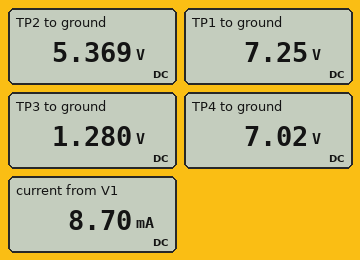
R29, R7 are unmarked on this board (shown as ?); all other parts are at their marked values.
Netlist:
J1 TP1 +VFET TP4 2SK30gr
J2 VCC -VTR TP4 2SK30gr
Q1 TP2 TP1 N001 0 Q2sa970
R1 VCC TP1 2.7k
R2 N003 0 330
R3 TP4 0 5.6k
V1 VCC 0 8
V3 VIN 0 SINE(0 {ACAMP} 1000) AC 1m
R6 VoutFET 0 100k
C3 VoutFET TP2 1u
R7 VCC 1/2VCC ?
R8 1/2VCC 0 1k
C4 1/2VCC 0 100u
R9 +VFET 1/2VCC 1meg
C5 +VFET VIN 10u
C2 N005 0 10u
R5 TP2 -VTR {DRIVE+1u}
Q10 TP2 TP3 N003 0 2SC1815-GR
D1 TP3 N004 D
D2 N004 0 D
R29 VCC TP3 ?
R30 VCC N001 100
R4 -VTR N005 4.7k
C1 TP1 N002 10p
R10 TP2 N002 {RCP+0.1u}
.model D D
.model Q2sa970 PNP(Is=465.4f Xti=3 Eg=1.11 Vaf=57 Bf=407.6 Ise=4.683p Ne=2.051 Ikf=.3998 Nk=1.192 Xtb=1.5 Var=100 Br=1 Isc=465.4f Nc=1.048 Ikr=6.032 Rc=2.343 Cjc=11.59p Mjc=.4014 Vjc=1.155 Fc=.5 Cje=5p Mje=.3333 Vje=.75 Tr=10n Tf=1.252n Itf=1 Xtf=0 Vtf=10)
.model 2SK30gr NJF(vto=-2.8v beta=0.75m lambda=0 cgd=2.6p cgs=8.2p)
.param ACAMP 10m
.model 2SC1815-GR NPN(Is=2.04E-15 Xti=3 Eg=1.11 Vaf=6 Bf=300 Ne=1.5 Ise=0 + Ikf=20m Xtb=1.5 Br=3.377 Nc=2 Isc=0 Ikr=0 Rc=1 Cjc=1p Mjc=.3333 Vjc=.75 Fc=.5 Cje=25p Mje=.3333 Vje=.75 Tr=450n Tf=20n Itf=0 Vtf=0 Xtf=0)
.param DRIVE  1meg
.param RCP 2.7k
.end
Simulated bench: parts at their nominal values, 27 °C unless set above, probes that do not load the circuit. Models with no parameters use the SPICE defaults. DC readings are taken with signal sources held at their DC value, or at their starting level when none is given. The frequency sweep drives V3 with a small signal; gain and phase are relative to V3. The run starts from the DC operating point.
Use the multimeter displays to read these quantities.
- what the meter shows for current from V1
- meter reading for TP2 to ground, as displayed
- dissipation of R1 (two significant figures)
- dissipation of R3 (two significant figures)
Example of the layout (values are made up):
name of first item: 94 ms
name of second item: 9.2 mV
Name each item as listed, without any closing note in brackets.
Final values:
what the meter shows for current from V1: 8.70 mA
meter reading for TP2 to ground, as displayed: 5.369 V
dissipation of R1: 210 µW
dissipation of R3: 8.8 mW
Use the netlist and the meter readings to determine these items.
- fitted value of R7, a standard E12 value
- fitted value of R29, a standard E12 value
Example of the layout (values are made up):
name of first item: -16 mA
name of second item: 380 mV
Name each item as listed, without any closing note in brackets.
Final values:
fitted value of R7, a standard E12 value: 560 Ω
fitted value of R29, a standard E12 value: 12 kΩ
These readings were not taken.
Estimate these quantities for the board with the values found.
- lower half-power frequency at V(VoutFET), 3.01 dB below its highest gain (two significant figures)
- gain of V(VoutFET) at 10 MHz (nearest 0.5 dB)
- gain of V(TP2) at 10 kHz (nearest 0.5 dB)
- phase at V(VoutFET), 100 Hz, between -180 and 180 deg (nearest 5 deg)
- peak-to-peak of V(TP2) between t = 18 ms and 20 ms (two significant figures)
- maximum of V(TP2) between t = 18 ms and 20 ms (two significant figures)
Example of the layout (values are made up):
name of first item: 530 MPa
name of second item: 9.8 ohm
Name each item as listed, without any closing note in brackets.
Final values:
lower half-power frequency at V(VoutFET), 3.01 dB below its highest gain: 2.3 Hz
gain of V(VoutFET) at 10 MHz: -8.5 dB
gain of V(TP2) at 10 kHz: 31.0 dB
phase at V(VoutFET), 100 Hz, between -180 and 180 deg: 0 deg
peak-to-peak of V(TP2) between t = 18 ms and 20 ms: 740 mV
maximum of V(TP2) between t = 18 ms and 20 ms: 5.7 V
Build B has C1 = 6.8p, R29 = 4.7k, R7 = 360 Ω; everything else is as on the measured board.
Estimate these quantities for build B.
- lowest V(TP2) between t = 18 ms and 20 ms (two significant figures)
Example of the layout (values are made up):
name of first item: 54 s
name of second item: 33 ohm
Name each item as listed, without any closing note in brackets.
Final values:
lowest V(TP2) between t = 18 ms and 20 ms: 5.4 V
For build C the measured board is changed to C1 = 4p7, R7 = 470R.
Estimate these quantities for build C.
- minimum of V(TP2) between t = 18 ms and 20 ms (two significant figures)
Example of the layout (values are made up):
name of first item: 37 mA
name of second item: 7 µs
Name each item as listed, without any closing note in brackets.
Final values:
minimum of V(TP2) between t = 18 ms and 20 ms: 5.2 V
